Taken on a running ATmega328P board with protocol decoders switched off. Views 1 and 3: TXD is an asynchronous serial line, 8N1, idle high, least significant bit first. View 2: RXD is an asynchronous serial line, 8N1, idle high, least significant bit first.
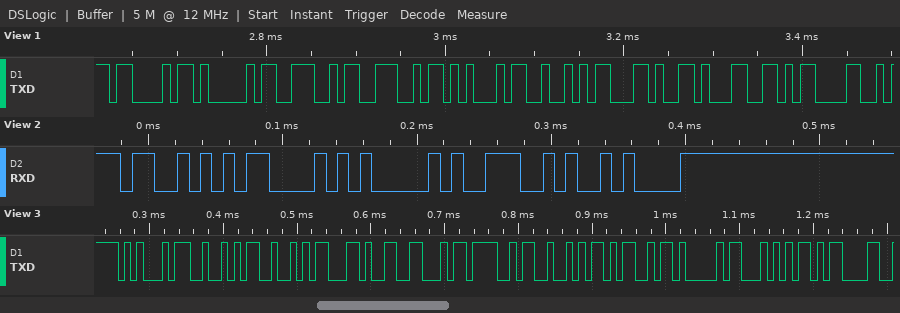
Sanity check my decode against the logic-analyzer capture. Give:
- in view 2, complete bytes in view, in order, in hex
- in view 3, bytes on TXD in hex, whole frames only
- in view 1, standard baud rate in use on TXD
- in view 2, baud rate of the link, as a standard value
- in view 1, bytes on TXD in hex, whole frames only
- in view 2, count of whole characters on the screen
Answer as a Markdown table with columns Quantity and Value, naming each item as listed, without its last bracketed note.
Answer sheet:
| Quantity | Value |
|---|---|
| in view 2, complete bytes in view, in order, in hex | 0x53 0x43 0x41 0x4E 0x0A |
| in view 3, bytes on TXD in hex, whole frames only | 45 52 52 2C 46 4F 52 4D 41 54 0D |
| in view 1, standard baud rate in use on TXD | 115200 baud |
| in view 2, baud rate of the link, as a standard value | 115200 baud |
| in view 1, bytes on TXD in hex, whole frames only | 43 41 4E 4E 45 52 2C 31 0D |
| in view 2, count of whole characters on the screen | 5 |
